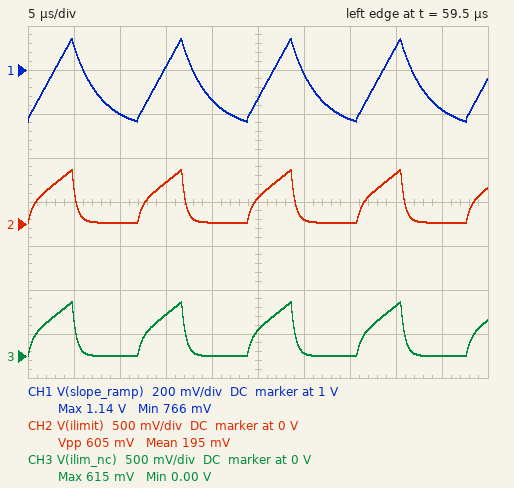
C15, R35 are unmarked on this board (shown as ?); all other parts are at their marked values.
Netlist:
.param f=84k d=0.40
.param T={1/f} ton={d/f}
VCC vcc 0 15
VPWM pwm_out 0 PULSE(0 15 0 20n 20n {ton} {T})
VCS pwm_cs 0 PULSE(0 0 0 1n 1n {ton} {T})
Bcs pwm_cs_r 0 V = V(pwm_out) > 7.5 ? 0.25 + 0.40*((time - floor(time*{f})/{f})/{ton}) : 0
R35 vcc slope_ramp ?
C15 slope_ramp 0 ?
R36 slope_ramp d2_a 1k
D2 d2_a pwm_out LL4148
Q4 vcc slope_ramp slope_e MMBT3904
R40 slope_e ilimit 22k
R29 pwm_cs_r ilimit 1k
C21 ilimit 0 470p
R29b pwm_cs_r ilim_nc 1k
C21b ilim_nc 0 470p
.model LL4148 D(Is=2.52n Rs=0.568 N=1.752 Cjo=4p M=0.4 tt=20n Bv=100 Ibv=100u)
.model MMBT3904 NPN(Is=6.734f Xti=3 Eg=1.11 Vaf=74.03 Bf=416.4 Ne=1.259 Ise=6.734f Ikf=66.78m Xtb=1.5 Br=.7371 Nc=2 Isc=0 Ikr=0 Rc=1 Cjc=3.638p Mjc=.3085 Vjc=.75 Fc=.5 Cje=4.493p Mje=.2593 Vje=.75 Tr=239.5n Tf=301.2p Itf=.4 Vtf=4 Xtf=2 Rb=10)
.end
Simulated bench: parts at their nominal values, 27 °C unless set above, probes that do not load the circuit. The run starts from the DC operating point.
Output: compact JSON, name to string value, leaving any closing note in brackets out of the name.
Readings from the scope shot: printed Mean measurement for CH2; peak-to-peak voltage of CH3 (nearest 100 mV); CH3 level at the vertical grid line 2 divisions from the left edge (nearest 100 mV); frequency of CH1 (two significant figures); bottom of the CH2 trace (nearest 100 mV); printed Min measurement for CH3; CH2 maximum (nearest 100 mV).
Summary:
{"printed Mean measurement for CH2": "195 mV", "peak-to-peak voltage of CH3": "600 mV", "CH3 level at the vertical grid line 2 divisions from the left edge": "0 V", "frequency of CH1": "84 kHz", "bottom of the CH2 trace": "0 V", "printed Min measurement for CH3": "0.00 V", "CH2 maximum": "600 mV"}
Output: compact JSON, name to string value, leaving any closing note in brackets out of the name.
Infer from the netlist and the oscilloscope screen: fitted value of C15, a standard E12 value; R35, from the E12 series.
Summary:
{"fitted value of C15, a standard E12 value": "2.7 nF", "R35, from the E12 series": "68 kΩ"}
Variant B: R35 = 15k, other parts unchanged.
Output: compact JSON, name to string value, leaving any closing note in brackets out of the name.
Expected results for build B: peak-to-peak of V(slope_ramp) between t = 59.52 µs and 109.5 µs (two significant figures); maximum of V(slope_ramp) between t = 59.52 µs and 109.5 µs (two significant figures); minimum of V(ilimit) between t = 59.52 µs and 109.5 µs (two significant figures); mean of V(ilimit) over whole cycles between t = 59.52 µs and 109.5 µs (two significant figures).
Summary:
{"peak-to-peak of V(slope_ramp) between t = 59.52 µs and 109.5 µs": "1.5 V", "maximum of V(slope_ramp) between t = 59.52 µs and 109.5 µs": "3.1 V", "minimum of V(ilimit) between t = 59.52 µs and 109.5 µs": "45 mV", "mean of V(ilimit) over whole cycles between t = 59.52 µs and 109.5 µs": "240 mV"}
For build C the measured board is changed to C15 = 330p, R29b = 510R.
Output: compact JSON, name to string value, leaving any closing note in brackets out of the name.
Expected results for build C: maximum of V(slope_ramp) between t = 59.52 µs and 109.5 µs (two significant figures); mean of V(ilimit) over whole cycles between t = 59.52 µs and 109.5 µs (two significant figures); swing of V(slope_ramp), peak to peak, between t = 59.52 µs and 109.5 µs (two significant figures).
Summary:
{"maximum of V(slope_ramp) between t = 59.52 µs and 109.5 µs": "3.5 V", "mean of V(ilimit) over whole cycles between t = 59.52 µs and 109.5 µs": "210 mV", "swing of V(slope_ramp), peak to peak, between t = 59.52 µs and 109.5 µs": "2.8 V"}
